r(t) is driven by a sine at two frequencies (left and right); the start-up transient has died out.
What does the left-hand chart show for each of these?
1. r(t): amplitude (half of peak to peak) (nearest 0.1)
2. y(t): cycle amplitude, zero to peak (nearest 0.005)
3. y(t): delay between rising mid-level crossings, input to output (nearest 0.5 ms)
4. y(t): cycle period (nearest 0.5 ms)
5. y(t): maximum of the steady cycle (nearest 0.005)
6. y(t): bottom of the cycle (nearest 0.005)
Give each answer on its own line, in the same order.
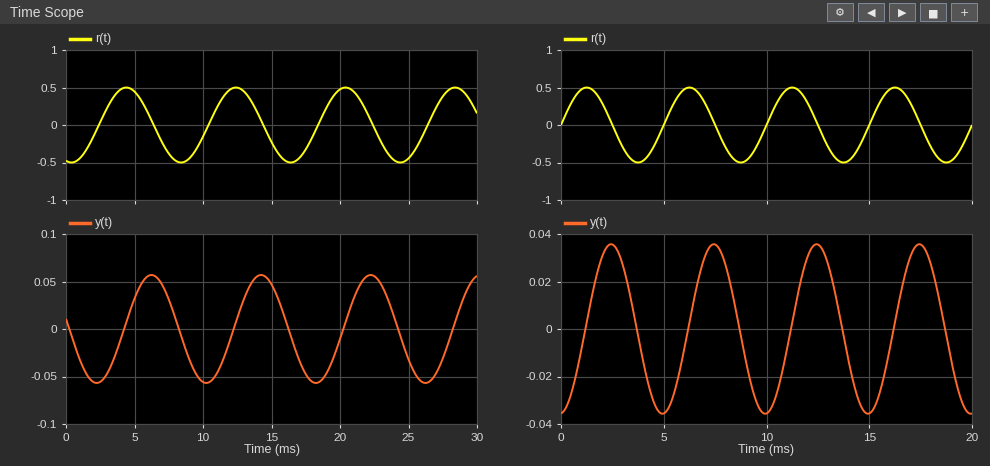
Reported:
0.5
0.055
2.0 ms
8.0 ms
0.055
-0.055
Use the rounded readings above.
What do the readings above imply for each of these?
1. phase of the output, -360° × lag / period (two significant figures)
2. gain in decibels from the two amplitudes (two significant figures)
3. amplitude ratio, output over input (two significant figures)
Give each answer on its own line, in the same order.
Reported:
-90°
-19 dB
0.11
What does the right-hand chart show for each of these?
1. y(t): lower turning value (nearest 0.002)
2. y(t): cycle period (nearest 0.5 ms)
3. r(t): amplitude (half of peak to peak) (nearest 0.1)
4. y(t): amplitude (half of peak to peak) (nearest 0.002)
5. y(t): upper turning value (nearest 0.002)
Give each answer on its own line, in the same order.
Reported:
-0.036
5.0 ms
0.5
0.036
0.036
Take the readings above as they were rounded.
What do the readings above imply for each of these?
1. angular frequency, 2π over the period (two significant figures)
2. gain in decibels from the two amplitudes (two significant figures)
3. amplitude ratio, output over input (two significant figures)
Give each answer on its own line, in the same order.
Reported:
1.3 rad/ms
-23 dB
0.072
